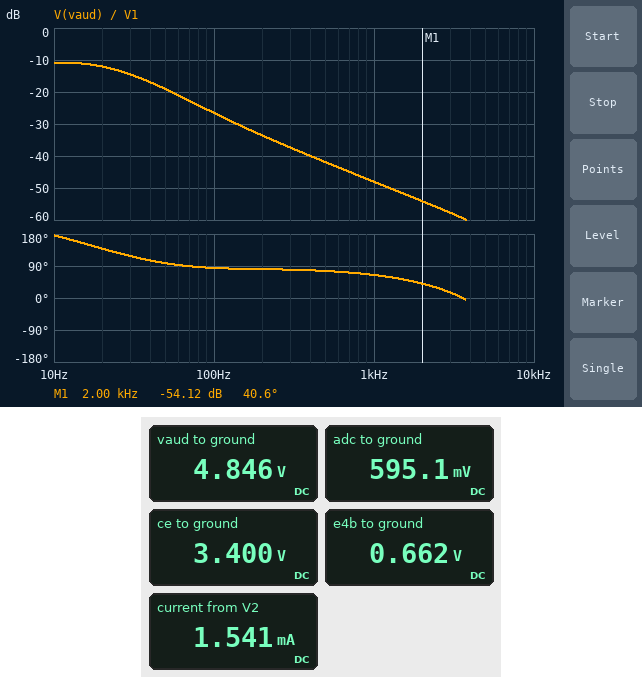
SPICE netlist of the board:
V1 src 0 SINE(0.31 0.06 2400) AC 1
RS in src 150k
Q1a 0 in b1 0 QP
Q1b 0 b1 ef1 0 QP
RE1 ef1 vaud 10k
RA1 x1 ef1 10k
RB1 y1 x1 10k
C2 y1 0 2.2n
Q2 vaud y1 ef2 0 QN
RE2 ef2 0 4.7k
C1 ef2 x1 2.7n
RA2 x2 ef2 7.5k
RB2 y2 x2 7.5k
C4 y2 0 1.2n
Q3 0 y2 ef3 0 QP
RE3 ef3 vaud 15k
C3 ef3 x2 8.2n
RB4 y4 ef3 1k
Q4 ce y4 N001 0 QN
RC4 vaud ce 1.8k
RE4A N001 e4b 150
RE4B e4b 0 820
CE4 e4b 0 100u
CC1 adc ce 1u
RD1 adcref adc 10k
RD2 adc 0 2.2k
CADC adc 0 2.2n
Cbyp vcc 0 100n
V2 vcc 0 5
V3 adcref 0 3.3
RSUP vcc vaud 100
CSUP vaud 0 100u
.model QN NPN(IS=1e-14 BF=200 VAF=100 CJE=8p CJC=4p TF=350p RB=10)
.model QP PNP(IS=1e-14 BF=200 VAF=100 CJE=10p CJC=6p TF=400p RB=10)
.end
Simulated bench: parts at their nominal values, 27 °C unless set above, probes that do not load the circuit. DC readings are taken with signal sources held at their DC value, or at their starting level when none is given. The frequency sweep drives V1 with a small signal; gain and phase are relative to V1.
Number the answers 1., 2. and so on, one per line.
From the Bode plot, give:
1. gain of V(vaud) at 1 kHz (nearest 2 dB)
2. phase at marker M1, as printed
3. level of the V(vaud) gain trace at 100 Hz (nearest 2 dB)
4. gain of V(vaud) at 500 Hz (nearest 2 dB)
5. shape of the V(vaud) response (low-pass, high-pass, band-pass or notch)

1. -48 dB
2. 40.6 deg
3. -26 dB
4. -42 dB
5. low-pass
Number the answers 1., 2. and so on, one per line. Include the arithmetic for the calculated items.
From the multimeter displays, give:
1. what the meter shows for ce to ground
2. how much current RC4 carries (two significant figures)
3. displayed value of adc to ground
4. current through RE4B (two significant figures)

1. 3.400 V
2. (4.846 V - 3.4 V) / 1.8 kΩ = 800 µA
3. 595.1 mV
4. (662 mV) / 820 Ω = 810 µA
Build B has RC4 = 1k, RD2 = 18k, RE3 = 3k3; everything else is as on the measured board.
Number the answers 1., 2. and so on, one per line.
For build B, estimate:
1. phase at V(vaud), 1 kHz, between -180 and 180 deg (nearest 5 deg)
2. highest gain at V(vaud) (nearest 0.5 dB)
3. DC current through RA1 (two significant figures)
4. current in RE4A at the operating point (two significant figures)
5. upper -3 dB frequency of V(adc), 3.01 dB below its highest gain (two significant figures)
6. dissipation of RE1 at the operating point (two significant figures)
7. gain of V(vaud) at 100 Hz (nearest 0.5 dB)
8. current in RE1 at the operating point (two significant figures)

1. 65 deg
2. -11.5 dB
3. 800 nA
4. 900 µA
5. 6.2 kHz
6. 1.1 mW
7. -24.0 dB
8. 330 µA
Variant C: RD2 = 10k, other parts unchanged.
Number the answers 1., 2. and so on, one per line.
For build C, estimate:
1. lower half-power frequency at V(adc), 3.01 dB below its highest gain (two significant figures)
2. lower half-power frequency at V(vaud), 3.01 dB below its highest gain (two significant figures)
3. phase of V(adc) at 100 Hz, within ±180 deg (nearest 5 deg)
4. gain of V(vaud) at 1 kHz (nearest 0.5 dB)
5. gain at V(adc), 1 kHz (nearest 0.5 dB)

1. 27 Hz
2. 4.4 Hz
3. -165 deg
4. -45.0 dB
5. 16.0 dB
